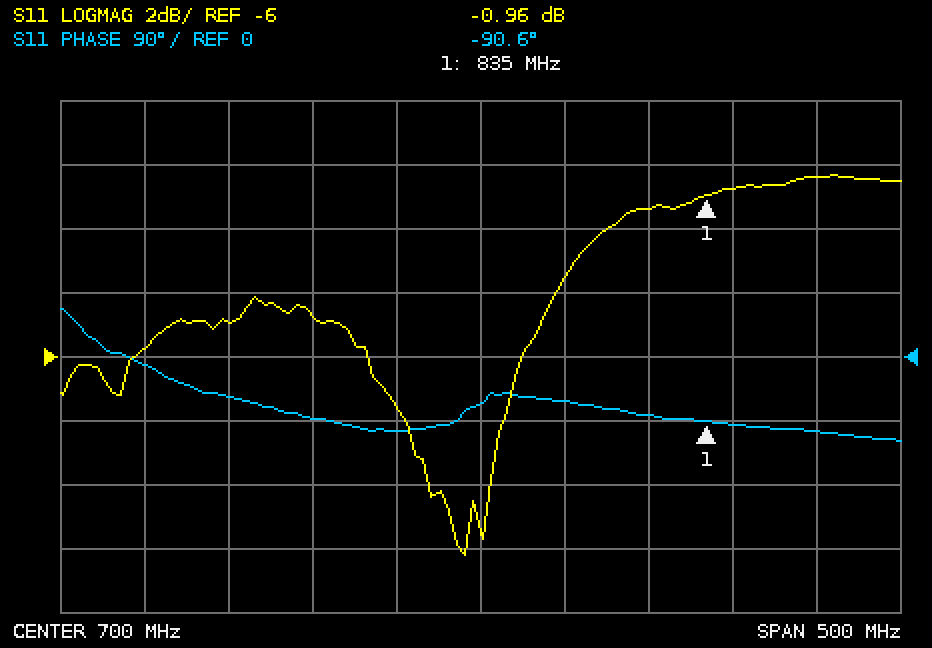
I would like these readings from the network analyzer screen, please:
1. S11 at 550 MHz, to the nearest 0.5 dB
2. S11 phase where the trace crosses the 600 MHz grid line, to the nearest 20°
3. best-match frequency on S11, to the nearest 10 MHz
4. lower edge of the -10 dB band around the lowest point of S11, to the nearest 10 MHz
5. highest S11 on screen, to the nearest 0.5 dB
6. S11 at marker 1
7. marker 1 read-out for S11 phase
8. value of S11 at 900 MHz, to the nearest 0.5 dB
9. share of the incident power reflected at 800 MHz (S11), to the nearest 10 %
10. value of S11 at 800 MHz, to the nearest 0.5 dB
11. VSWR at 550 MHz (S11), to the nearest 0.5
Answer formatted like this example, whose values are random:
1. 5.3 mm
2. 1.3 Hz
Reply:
1. -5.0 dB
2. -80°
3. 690 MHz
4. 670 MHz
5. -0.5 dB
6. -0.96 dB
7. -90.6°
8. -0.5 dB
9. 70 %
10. -1.5 dB
11. 3.5
